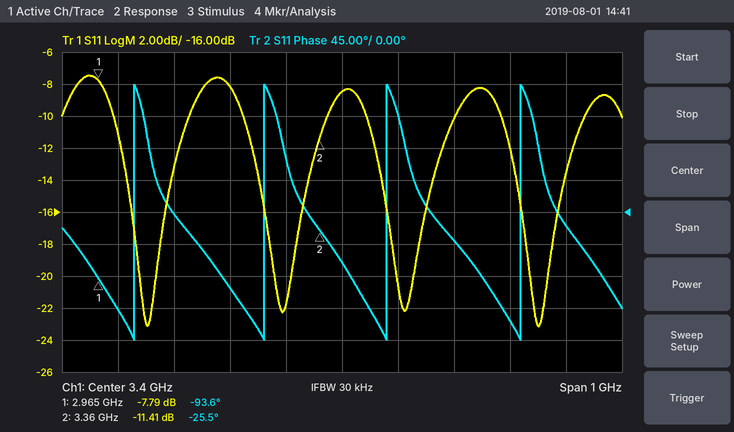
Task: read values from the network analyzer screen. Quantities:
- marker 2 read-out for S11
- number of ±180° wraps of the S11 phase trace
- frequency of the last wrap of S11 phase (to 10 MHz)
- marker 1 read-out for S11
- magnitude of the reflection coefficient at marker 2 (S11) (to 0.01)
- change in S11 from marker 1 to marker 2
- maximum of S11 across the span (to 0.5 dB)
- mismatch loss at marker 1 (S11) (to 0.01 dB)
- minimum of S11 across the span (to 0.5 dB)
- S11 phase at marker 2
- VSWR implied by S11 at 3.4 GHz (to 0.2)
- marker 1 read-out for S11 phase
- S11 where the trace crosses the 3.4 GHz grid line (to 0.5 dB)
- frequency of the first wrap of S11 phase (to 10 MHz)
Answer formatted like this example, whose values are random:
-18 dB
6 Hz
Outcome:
-11.41 dB
4
3.72 GHz
-7.79 dB
0.27
-3.62 dB
-7.5 dB
0.79 dB
-23.0 dB
-25.5°
2.2
-93.6°
-8.5 dB
3.03 GHz
